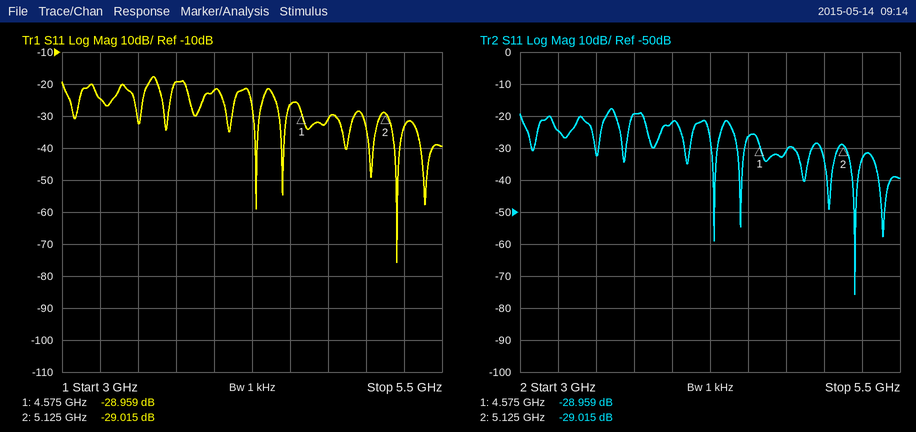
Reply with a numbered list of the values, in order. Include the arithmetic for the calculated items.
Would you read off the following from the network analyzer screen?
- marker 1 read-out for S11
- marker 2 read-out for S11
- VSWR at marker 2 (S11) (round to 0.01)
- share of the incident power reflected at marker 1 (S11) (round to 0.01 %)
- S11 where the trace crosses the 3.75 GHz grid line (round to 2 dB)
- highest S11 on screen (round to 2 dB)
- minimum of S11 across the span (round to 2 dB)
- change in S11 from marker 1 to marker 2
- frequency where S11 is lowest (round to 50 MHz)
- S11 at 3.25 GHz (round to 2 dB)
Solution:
1. -28.959 dB
2. -29.015 dB
3. (1 + 0.0354)/(1 − 0.0354) ≈ 1.07
4. 10^(-28.959/10) ≈ 0.13 %
5. -20 dB
6. -18 dB
7. -76 dB
8. -29.015 − (-28.959) = -0.056 dB
9. 5.20 GHz
10. -24 dB
